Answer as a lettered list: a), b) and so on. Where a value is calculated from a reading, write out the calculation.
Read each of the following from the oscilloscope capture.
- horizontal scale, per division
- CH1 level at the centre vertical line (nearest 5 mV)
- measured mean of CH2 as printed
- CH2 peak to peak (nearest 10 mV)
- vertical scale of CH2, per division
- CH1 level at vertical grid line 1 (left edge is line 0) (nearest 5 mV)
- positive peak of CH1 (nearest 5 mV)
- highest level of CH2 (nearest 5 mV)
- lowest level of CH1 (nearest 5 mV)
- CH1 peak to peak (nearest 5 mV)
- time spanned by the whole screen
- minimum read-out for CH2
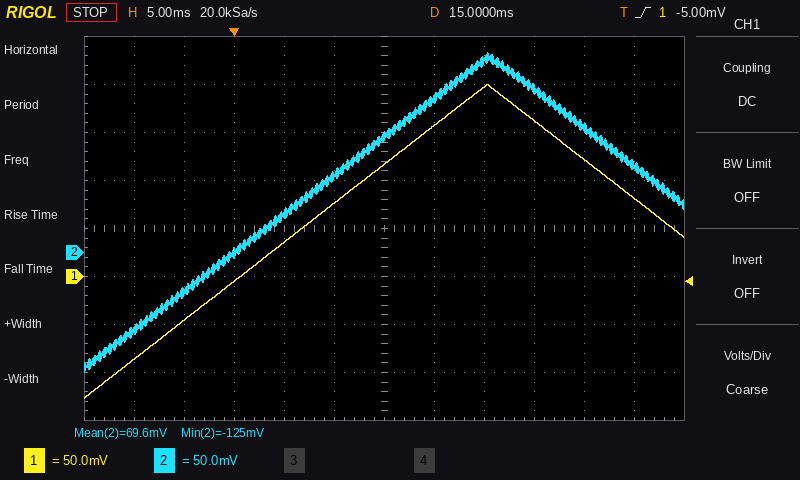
a) 5 ms
b) 115 mV
c) 69.6 mV
d) 330 mV
e) 50 mV
f) -85 mV
g) 200 mV
h) 210 mV
i) -125 mV
j) 200 mV − (-125 mV) = 325 mV
k) 60 ms
l) -125 mV
